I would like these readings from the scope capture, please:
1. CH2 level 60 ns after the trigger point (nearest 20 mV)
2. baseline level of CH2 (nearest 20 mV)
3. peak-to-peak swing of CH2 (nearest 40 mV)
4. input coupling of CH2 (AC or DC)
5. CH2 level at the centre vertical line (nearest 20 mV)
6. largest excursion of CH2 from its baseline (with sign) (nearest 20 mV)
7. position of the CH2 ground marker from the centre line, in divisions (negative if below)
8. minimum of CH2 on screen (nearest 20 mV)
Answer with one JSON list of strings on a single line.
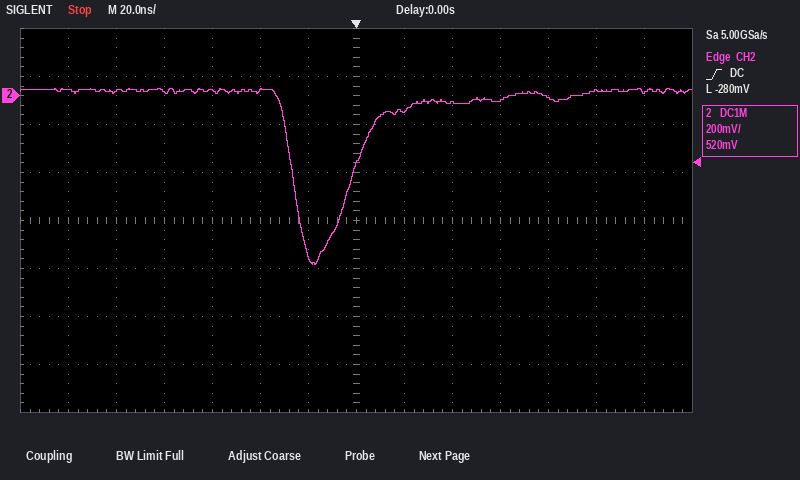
["-20 mV", "20 mV", "720 mV", "DC", "-280 mV", "-720 mV", "+2.6 div", "-700 mV"]
